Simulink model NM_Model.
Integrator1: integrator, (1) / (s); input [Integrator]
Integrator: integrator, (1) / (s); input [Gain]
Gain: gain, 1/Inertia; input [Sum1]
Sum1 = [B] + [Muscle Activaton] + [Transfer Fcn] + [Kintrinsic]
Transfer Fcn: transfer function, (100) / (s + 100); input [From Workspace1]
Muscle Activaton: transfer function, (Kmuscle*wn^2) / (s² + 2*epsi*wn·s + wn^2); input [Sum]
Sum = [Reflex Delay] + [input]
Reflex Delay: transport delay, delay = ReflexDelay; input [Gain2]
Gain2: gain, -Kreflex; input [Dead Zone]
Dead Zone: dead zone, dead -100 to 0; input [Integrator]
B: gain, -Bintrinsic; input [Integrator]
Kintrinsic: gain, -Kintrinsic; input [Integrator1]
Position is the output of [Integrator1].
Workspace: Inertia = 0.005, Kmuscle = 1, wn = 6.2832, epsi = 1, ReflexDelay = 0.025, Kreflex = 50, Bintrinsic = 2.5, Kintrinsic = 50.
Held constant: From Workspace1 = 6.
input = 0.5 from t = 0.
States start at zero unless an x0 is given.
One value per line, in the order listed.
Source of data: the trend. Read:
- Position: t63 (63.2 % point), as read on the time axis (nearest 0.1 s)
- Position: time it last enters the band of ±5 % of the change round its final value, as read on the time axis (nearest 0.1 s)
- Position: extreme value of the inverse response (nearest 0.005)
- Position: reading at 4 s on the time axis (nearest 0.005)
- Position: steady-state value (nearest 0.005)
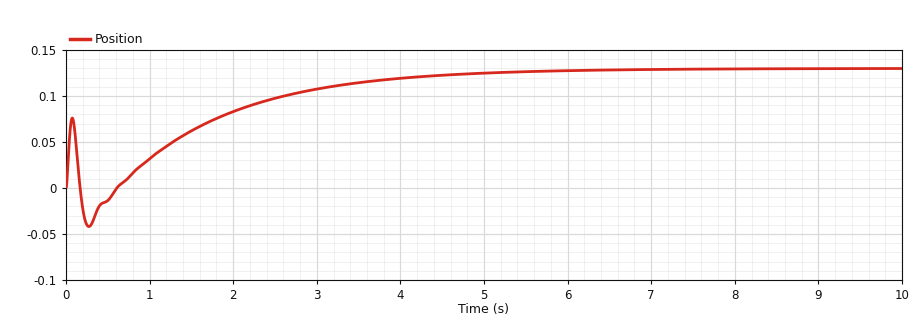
2.0 s
4.7 s
-0.040
0.120
0.130
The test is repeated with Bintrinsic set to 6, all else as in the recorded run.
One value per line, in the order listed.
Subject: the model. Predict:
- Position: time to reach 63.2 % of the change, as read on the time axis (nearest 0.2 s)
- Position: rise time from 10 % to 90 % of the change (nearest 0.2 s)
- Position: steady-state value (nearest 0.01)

1.6 s
3.4 s
0.13
